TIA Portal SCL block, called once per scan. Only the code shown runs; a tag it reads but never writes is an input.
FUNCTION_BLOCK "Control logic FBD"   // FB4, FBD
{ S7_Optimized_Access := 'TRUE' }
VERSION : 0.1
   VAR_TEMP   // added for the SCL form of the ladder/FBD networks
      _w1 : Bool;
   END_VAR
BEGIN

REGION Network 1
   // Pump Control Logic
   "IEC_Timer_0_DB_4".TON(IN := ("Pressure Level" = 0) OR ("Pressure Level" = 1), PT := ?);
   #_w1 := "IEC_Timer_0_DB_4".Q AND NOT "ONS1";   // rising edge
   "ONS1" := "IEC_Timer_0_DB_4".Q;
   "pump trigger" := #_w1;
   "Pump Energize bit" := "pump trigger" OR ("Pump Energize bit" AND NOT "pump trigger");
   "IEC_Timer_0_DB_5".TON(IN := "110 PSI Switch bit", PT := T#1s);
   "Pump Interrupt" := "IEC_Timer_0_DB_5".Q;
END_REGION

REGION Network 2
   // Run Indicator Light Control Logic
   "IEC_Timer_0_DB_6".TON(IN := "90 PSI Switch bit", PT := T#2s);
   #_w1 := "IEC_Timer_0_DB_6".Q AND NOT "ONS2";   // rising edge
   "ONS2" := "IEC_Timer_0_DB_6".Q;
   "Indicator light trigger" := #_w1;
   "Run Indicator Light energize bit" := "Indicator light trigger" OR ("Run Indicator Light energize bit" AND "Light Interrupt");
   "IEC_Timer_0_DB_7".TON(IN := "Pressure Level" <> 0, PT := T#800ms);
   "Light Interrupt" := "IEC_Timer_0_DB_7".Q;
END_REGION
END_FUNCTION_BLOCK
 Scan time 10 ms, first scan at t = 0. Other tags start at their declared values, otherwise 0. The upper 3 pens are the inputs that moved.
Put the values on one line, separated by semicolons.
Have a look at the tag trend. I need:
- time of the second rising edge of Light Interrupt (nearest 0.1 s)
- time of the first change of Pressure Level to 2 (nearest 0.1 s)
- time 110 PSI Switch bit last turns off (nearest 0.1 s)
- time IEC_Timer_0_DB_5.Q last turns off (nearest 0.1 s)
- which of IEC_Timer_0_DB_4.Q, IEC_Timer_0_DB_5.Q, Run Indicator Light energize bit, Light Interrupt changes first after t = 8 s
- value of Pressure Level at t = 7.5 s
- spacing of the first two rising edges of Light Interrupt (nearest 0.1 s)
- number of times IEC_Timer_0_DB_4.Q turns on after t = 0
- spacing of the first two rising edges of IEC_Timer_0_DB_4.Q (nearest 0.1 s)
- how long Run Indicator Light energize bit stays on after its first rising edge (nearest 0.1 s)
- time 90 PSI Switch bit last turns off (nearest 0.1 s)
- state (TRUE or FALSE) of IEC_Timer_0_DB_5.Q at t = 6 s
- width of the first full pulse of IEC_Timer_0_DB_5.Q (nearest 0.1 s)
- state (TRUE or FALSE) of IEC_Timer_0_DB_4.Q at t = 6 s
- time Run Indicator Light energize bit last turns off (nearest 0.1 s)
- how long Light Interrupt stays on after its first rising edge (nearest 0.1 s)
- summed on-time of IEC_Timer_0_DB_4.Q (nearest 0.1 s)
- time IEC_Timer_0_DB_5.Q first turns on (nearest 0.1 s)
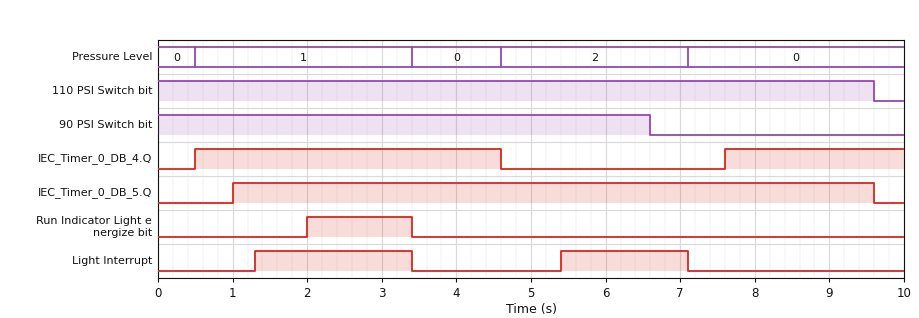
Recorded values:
5.4 s; 4.6 s; 9.6 s; 9.6 s; IEC_Timer_0_DB_5.Q; 0; 4.1 s; 2; 7.1 s; 1.4 s; 6.6 s; TRUE; 8.6 s; FALSE; 3.4 s; 2.1 s; 6.5 s; 1.0 s
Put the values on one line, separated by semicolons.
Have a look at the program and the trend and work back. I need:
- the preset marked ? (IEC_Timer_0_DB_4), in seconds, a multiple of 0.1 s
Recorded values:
0.5 s
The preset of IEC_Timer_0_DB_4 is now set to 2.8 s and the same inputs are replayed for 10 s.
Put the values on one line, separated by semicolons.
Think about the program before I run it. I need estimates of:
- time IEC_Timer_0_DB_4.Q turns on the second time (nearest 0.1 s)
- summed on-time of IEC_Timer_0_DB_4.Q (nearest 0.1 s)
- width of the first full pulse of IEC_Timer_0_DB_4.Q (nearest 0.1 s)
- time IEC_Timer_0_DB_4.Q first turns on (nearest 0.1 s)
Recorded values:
9.9 s; 1.9 s; 1.8 s; 2.8 s
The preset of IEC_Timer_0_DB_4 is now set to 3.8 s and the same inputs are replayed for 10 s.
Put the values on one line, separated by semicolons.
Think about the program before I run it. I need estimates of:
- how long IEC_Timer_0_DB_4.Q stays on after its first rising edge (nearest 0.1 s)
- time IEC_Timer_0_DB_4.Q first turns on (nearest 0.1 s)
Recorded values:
0.8 s; 3.8 s
